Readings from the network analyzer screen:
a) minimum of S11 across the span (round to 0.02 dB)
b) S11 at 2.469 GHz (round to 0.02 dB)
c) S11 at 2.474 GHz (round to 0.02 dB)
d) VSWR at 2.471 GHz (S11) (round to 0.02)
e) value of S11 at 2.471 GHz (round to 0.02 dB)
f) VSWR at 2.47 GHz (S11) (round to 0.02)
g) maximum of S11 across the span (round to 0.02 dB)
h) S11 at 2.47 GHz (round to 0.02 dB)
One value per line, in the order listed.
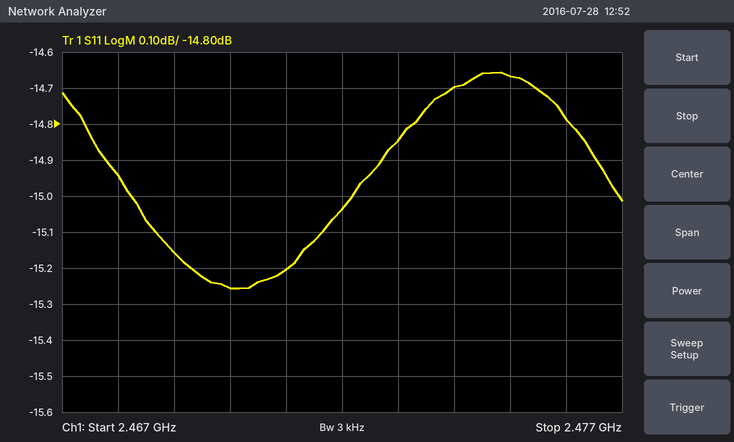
-15.26 dB
-15.16 dB
-14.70 dB
1.42
-15.20 dB
1.42
-14.66 dB
-15.26 dB
